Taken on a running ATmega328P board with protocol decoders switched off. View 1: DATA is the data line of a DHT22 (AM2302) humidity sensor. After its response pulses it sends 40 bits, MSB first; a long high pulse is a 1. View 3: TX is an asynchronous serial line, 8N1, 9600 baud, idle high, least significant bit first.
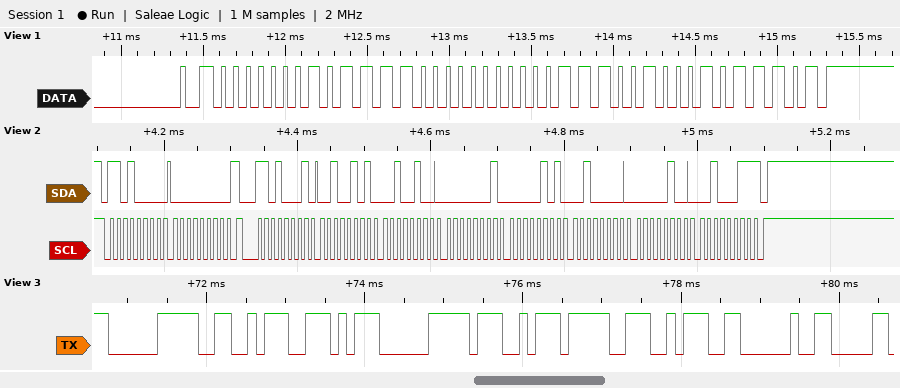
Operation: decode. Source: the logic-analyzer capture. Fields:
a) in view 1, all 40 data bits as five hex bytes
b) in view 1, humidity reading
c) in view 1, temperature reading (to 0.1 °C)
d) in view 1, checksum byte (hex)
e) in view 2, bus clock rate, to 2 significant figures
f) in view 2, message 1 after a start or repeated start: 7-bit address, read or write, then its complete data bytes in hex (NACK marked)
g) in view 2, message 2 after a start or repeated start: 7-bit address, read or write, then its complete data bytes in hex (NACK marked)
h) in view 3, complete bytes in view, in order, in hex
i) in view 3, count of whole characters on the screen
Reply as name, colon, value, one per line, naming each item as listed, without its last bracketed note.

in view 1, all 40 data bits as five hex bytes: 01 78 00 E4 5D
in view 1, humidity reading: 37.6 %
in view 1, temperature reading: 22.8 °C
in view 1, checksum byte: 0x5D
in view 2, bus clock rate, to 2 significant figures: 100 kHz
in view 2, message 1 after a start or repeated start: 7-bit address, read or write, then its complete data bytes in hex: 0x68 write: 00
in view 2, message 2 after a start or repeated start: 7-bit address, read or write, then its complete data bytes in hex: 0x68 read: 25 24 01 05 20 04 23 NACK
in view 3, complete bytes in view, in order, in hex: 0xE0 0xA6 0xAE 0xE0 0xA7 0x9F 0x3A 0x20
in view 3, count of whole characters on the screen: 8
